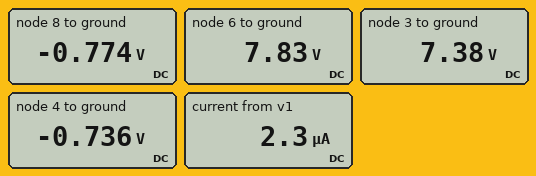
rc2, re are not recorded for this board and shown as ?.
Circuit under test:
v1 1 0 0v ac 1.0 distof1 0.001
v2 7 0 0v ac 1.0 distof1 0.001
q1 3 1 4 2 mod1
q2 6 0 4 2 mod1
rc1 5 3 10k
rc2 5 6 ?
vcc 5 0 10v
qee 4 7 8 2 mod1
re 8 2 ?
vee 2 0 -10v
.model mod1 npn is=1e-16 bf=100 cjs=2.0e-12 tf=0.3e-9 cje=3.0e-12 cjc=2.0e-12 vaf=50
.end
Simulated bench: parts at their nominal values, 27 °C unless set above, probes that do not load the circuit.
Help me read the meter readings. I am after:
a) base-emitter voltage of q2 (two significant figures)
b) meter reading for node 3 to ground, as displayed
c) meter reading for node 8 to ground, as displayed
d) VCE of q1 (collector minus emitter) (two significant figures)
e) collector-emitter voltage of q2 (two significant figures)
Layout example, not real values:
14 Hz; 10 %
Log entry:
740 mV; 7.38 V; -0.774 V; 8.1 V; 8.6 V
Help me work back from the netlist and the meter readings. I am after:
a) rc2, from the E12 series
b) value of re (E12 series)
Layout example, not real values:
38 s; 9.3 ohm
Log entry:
8.2 kΩ; 12 kΩ
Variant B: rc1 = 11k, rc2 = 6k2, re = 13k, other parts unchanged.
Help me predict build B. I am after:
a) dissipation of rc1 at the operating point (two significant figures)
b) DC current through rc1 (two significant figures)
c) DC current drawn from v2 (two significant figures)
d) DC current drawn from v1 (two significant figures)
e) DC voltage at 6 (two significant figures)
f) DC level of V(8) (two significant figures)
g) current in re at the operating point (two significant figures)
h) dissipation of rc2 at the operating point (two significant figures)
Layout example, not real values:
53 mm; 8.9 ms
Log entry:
640 µW; 240 µA; 220 µA; 2.1 µA; 8.5 V; -770 mV; 710 µA; 370 µW
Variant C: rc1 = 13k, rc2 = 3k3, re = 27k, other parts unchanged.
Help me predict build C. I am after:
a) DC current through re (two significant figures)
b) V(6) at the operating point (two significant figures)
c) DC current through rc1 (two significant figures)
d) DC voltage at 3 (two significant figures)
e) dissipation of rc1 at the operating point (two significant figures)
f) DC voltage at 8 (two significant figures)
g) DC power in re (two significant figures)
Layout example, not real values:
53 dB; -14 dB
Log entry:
340 µA; 9.6 V; 120 µA; 8.5 V; 180 µW; -750 mV; 3.2 mW
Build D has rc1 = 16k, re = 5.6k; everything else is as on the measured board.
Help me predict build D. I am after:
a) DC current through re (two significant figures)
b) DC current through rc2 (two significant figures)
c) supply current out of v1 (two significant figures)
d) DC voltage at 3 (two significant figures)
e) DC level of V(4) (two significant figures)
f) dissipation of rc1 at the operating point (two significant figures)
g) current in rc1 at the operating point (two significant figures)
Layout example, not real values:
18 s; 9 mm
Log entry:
1.6 mA; 570 µA; 5.1 µA; 1.5 V; -760 mV; 4.5 mW; 530 µA
